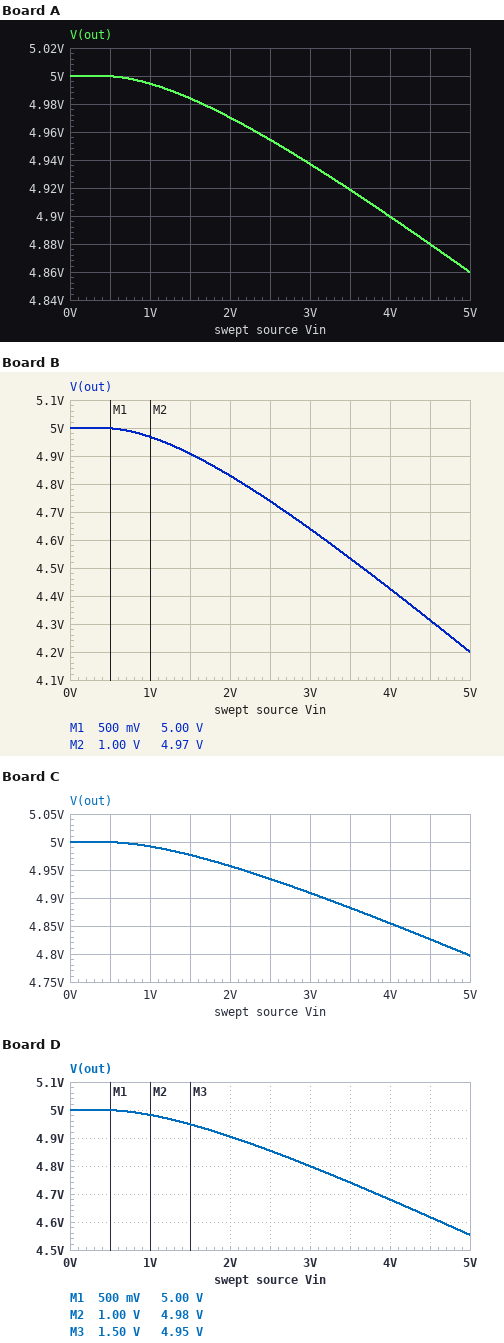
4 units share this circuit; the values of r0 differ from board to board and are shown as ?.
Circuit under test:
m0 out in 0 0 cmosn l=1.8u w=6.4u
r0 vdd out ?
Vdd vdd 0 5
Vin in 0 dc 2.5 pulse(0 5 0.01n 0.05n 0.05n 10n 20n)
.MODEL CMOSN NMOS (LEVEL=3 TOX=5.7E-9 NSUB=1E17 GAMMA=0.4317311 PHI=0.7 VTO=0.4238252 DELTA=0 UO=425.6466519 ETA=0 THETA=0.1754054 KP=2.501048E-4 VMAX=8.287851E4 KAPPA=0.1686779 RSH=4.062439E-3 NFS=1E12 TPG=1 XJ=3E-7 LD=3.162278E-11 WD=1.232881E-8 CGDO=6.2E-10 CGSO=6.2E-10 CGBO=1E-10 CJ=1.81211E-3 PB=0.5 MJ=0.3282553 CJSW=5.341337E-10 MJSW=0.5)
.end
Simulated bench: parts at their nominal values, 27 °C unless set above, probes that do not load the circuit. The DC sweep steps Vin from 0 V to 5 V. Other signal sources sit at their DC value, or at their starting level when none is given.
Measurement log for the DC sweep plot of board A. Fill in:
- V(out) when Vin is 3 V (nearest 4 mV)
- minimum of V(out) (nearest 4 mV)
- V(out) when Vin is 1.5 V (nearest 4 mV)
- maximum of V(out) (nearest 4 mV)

4.936 V
4.860 V
4.984 V
5.000 V
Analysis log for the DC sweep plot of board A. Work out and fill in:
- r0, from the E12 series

47 Ω
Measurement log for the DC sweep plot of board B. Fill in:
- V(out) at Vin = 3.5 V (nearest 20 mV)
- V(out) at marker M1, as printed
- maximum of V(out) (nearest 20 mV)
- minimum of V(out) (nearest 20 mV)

4.54 V
5.00 V
5.00 V
4.20 V
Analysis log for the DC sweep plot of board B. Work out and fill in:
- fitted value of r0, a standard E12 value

270 Ω
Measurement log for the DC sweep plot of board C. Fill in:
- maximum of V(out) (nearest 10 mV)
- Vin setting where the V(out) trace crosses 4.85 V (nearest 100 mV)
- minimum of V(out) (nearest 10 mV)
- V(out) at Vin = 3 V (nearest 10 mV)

5.00 V
4.1 V
4.80 V
4.91 V
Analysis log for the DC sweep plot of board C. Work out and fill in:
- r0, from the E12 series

68 Ω
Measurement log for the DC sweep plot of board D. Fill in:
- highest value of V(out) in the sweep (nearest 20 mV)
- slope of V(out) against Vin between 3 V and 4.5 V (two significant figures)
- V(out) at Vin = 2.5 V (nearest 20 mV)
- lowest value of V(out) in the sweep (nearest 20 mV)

5.00 V
-0.12 V/V
4.86 V
4.56 V
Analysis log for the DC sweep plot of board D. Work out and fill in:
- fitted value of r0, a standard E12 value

150 Ω
